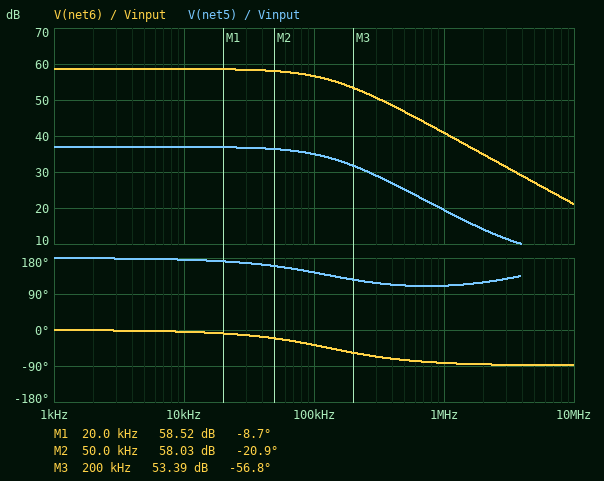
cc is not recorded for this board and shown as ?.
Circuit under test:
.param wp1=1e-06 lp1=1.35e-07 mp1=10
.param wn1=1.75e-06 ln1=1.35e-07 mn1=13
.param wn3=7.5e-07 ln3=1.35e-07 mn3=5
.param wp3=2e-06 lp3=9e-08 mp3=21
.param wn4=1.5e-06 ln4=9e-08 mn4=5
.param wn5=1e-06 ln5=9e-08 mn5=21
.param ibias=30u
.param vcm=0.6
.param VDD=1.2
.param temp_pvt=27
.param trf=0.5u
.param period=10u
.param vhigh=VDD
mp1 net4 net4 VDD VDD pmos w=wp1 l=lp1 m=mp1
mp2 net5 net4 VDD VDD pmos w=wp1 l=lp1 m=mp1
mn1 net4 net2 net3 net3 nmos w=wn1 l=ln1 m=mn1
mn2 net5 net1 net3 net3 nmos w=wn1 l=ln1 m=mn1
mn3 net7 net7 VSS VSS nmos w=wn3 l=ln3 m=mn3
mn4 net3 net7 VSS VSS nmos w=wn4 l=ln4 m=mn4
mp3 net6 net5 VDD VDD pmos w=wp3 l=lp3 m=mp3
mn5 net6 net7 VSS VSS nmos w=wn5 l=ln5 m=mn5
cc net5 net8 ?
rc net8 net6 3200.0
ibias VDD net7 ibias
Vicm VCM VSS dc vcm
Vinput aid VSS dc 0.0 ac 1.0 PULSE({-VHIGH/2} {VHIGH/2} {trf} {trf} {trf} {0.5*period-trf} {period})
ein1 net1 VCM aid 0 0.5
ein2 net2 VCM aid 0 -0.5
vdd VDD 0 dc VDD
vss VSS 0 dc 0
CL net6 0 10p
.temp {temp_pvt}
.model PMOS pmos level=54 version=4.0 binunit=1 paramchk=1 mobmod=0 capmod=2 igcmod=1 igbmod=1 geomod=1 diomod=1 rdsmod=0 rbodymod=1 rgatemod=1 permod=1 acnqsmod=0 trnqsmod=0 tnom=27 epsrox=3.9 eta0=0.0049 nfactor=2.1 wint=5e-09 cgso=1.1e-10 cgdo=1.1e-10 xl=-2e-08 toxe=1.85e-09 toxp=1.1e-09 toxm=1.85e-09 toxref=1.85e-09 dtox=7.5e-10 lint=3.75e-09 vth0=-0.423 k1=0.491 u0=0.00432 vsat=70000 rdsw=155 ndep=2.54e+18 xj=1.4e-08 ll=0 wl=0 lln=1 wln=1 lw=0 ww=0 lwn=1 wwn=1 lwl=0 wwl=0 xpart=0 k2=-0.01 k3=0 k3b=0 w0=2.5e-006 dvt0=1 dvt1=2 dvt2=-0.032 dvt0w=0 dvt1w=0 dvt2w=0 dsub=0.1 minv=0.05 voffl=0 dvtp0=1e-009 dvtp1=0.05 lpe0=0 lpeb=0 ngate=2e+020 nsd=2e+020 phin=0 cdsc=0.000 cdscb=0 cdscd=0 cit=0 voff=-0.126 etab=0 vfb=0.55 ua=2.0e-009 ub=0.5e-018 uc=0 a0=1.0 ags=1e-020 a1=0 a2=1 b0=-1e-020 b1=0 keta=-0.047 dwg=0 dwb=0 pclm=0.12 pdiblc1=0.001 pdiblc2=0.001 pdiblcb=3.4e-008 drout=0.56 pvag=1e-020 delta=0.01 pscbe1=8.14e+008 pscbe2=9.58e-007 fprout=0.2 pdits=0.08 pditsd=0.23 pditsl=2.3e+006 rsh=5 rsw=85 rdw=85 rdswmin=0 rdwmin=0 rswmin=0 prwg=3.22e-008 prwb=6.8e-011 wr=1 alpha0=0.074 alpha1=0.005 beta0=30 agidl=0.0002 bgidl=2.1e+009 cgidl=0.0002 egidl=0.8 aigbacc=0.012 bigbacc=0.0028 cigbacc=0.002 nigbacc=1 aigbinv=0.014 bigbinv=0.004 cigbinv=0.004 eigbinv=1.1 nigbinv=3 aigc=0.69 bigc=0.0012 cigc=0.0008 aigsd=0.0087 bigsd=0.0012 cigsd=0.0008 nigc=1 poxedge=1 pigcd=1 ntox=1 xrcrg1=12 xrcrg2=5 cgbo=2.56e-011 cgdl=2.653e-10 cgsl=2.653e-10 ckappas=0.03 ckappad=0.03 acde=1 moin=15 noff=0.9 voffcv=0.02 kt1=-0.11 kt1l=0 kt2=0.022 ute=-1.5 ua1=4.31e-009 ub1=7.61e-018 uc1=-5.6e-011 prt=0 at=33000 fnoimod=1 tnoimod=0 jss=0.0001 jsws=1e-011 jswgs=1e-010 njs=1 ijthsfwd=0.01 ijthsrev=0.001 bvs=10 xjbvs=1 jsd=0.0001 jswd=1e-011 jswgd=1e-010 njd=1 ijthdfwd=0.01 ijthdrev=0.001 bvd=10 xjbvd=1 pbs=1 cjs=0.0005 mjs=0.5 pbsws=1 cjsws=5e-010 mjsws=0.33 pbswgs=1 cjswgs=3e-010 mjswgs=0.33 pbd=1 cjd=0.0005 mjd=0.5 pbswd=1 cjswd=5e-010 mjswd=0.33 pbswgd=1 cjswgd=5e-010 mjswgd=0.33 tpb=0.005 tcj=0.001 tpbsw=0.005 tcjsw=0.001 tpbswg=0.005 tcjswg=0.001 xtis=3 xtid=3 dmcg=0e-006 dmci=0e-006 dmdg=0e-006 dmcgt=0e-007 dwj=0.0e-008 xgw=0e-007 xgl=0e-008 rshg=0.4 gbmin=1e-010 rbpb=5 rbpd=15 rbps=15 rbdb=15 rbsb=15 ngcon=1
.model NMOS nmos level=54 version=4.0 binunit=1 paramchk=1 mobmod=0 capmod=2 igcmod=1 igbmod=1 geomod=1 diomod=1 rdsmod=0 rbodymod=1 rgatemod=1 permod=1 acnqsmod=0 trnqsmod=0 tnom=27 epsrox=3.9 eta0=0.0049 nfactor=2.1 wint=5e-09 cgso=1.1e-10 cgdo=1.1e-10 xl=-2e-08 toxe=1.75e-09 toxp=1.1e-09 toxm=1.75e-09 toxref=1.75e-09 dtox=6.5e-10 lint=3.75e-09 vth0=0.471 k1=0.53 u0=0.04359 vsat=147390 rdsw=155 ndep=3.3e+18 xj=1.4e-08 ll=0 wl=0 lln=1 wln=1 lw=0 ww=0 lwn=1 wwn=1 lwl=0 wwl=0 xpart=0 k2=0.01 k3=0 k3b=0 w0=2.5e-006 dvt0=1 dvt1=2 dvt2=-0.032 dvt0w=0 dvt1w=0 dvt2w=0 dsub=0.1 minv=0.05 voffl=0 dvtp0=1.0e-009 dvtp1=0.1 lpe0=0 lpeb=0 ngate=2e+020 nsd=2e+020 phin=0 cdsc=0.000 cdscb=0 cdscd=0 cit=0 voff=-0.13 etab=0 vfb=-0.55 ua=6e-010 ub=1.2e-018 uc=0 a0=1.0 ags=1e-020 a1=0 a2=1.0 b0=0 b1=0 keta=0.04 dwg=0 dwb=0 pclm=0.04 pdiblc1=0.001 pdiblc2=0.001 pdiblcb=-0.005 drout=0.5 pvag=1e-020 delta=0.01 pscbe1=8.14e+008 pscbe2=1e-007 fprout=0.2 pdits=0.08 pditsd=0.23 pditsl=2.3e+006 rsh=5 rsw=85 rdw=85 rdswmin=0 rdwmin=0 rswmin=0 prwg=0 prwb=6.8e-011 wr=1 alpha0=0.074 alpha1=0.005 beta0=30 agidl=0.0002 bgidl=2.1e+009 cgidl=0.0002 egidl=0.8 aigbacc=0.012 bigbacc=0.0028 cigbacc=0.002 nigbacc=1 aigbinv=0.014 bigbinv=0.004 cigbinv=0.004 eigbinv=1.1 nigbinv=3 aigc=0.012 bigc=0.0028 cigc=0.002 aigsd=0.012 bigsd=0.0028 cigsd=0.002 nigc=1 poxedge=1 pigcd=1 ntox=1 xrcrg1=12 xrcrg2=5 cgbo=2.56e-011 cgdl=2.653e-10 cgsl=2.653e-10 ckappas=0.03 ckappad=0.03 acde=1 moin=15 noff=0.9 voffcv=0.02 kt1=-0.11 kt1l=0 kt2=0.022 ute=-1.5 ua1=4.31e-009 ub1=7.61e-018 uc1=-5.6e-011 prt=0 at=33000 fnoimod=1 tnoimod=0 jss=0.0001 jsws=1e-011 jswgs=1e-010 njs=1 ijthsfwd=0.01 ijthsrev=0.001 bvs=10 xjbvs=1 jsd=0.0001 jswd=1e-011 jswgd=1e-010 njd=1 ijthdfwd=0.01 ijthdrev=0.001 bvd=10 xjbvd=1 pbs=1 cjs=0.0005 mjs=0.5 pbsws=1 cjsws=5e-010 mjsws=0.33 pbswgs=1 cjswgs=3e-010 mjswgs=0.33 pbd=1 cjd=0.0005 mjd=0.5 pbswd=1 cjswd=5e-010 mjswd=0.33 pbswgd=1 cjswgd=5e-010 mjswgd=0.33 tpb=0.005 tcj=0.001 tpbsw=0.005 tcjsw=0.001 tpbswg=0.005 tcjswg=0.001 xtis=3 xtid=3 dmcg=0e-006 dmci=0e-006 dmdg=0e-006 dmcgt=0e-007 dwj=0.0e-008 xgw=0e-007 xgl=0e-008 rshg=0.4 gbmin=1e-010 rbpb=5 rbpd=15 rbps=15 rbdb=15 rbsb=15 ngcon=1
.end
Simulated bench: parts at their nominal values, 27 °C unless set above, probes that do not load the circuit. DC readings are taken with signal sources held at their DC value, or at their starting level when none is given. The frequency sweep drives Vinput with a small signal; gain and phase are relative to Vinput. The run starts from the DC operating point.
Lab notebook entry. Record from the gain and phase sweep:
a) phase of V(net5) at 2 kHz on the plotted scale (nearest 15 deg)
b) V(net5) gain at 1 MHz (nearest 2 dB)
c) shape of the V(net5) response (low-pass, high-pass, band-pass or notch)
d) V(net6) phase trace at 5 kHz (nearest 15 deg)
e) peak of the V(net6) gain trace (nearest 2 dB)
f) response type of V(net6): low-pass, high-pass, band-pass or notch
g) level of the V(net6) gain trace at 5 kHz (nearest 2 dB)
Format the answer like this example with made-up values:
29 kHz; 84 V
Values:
180 deg; 20 dB; low-pass; 0 deg; 58 dB; low-pass; 58 dB
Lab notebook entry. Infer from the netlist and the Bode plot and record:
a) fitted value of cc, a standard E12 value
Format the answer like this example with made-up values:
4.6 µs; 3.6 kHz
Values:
1.2 pF
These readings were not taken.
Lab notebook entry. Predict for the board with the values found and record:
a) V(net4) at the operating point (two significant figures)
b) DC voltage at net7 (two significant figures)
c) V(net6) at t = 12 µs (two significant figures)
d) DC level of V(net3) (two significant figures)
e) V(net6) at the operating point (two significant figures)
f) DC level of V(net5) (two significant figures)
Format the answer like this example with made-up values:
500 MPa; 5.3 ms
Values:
640 mV; 470 mV; 1.2 V; 200 mV; 980 mV; 640 mV
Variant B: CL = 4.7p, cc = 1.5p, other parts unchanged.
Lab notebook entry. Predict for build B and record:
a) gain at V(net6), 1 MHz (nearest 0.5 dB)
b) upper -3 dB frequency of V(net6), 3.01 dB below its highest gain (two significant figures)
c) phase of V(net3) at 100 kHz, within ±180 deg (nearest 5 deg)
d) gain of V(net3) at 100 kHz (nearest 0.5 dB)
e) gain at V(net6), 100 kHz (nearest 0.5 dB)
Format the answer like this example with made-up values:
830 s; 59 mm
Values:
39.0 dB; 110 kHz; 140 deg; -13.0 dB; 56.0 dB
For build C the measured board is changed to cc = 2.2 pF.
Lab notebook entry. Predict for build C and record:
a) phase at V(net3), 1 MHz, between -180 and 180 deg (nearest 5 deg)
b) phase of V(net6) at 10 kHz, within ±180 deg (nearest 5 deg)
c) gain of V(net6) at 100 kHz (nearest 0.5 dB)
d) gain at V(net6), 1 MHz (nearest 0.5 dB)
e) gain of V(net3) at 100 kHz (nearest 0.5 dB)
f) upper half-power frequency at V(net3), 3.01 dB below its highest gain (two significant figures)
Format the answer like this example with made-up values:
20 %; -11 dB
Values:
110 deg; -10 deg; 54.0 dB; 36.0 dB; -15.0 dB; 73 kHz
